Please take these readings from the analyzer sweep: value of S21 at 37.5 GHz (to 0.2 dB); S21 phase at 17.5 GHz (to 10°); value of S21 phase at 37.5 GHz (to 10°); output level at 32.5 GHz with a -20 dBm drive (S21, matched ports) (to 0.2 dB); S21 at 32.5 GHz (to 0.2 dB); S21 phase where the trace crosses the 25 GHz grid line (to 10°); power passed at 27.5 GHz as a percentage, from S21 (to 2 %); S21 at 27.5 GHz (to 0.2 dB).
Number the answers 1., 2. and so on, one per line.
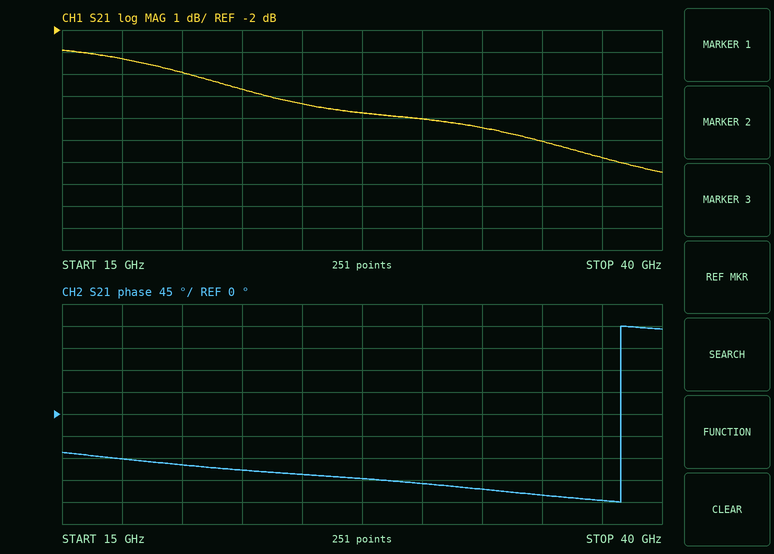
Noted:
1. -7.8 dB
2. -90°
3. -180°
4. -26.4 dBm
5. -6.4 dB
6. -120°
7. 26 %
8. -5.8 dB
